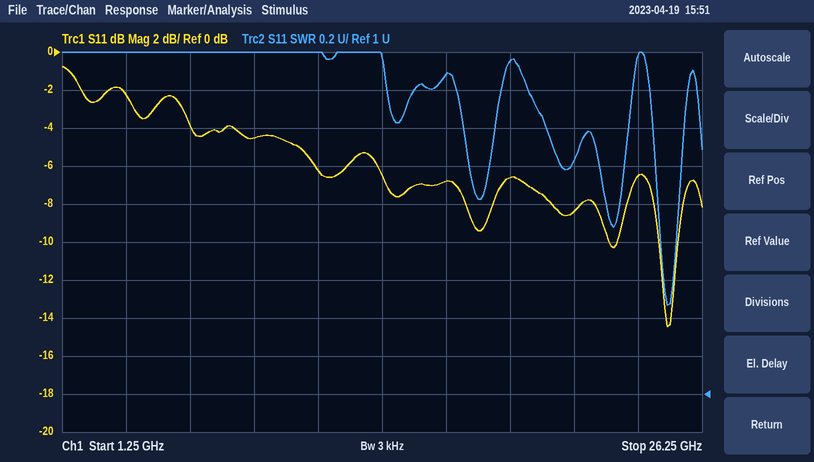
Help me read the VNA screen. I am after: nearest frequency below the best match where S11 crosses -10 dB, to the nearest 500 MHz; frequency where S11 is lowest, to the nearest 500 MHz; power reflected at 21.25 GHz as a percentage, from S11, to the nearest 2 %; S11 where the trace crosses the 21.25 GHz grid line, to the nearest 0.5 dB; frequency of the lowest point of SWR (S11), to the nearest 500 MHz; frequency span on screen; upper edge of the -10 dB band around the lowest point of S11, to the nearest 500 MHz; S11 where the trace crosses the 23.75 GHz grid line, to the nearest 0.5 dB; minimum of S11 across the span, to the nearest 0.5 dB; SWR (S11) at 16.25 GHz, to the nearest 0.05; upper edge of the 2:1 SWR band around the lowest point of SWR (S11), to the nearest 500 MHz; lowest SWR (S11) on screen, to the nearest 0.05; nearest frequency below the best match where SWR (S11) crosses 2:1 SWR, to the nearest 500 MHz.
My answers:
24.5 GHz
25.0 GHz
14 %
-8.5 dB
25.0 GHz
25 GHz
25.5 GHz
-6.5 dB
-14.5 dB
2.70
25.5 GHz
1.45
24.5 GHz
